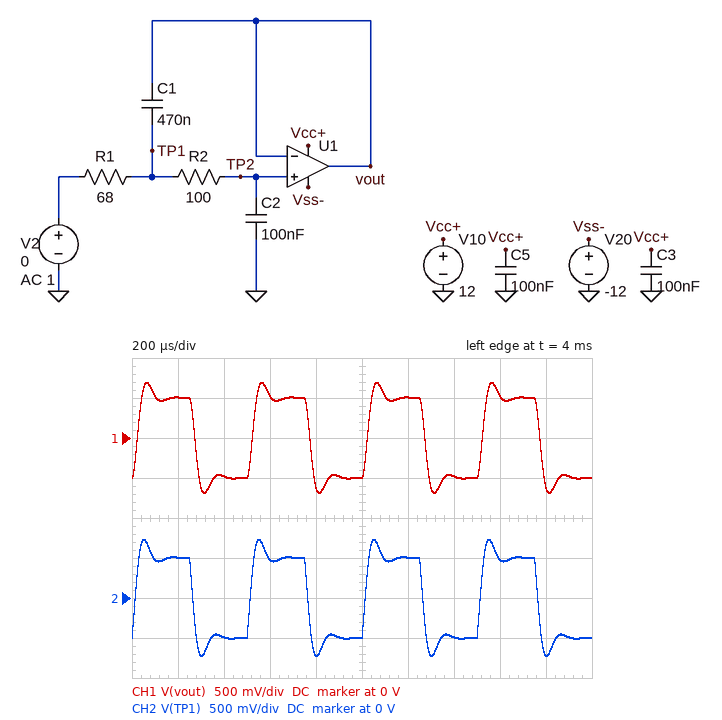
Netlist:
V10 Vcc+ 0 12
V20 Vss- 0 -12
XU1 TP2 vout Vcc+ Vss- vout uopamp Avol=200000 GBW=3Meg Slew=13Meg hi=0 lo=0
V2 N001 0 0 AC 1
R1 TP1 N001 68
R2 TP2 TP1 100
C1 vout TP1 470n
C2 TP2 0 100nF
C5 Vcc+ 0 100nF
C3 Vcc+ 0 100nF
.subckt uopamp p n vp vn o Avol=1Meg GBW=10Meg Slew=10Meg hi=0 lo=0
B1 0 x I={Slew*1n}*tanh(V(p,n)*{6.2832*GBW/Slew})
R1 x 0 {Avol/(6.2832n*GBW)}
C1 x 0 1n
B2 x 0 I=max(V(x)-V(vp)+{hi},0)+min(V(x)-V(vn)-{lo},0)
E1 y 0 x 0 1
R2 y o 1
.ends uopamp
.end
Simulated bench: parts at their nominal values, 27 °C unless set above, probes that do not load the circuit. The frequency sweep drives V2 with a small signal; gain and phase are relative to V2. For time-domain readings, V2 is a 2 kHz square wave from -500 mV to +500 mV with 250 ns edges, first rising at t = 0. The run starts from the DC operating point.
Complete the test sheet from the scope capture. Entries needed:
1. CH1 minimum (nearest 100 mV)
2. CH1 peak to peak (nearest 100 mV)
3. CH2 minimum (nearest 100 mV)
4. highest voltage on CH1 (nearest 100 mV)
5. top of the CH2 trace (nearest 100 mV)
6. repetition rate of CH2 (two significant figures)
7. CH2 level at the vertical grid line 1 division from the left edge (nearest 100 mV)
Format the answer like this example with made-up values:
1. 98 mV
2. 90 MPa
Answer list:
1. -700 mV
2. 1.4 V
3. -700 mV
4. 700 mV
5. 700 mV
6. 2.0 kHz
7. 500 mV
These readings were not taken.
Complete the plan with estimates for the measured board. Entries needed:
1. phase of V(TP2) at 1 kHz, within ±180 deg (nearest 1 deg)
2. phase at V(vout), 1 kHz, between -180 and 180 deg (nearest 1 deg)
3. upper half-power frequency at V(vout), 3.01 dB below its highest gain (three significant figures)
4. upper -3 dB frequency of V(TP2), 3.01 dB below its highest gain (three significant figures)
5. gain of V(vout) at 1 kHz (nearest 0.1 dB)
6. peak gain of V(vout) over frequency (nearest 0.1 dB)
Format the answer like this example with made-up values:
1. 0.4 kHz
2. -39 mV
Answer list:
1. -6 deg
2. -6 deg
3. 10.5 kHz
4. 10.5 kHz
5. 0.1 dB
6. 1.6 dB
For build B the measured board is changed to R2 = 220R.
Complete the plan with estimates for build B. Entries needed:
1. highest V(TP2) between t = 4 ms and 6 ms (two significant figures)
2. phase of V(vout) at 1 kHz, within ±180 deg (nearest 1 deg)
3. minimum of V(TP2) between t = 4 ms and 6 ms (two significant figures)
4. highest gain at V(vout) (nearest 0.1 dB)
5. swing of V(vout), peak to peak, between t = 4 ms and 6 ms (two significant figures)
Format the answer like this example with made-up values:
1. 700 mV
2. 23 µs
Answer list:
1. 630 mV
2. -11 deg
3. -630 mV
4. 0.8 dB
5. 1.3 V
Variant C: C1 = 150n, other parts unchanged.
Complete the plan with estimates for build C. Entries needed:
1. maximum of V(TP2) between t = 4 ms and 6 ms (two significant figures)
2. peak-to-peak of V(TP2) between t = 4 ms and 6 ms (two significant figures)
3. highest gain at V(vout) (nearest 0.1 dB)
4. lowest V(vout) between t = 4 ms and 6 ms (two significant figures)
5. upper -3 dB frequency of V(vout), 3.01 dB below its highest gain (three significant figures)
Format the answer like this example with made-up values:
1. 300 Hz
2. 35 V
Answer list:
1. 510 mV
2. 1.0 V
3. 0 dB
4. -510 mV
5. 13.1 kHz
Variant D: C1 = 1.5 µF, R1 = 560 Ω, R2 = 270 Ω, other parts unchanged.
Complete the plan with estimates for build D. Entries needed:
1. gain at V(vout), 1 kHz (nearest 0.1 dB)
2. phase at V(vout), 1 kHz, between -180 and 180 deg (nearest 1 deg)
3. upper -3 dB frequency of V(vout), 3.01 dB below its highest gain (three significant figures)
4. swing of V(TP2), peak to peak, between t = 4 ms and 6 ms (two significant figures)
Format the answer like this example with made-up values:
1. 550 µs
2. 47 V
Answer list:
1. 5.5 dB
2. -79 deg
3. 1.24 kHz
4. 450 mV
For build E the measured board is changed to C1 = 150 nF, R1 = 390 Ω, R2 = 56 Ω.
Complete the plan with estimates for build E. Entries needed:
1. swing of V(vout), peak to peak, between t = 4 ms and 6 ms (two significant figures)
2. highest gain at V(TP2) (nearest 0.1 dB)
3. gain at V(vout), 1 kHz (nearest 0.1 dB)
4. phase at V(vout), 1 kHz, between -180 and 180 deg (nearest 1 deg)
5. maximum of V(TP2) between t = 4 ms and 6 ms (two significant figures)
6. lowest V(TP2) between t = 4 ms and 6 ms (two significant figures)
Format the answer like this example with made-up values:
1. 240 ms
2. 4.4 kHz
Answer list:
1. 1.0 V
2. 0 dB
3. -0.2 dB
4. -16 deg
5. 500 mV
6. -500 mV
